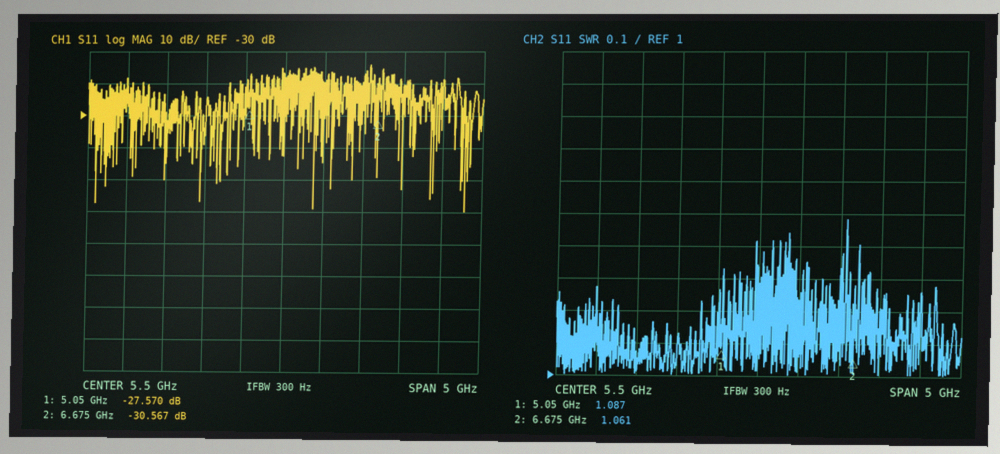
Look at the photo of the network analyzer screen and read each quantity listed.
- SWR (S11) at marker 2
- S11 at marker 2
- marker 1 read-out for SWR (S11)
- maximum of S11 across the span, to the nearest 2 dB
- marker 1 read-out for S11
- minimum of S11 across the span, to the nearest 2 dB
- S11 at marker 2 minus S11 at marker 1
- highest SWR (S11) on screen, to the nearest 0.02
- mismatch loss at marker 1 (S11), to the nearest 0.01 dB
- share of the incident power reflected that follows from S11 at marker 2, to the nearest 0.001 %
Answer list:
1.061
-30.567 dB
1.087
-14 dB
-27.570 dB
-60 dB
-2.997 dB
1.48
0.01 dB
0.088 %
